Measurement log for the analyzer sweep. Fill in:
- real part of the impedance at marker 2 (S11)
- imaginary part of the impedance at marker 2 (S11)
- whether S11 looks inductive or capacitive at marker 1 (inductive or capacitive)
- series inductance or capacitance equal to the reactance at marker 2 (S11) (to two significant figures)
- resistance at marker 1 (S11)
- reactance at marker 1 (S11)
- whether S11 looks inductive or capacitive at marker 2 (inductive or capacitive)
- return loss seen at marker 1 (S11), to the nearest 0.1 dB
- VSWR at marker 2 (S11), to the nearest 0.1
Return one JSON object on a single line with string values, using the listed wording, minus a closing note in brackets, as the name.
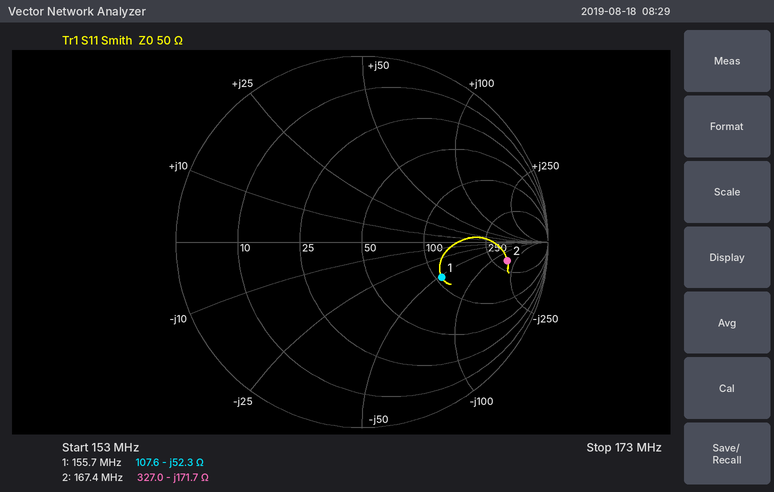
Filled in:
{"real part of the impedance at marker 2": "327.0 Ω", "imaginary part of the impedance at marker 2": "-171.7 Ω", "whether S11 looks inductive or capacitive at marker 1": "capacitive", "series inductance or capacitance equal to the reactance at marker 2 (S11)": "5.5 pF", "resistance at marker 1": "107.6 Ω", "reactance at marker 1": "-52.3 Ω", "whether S11 looks inductive or capacitive at marker 2": "capacitive", "return loss seen at marker 1 (S11), to the nearest 0.1 dB": "6.6 dB", "VSWR at marker 2 (S11), to the nearest 0.1": "8.4"}
